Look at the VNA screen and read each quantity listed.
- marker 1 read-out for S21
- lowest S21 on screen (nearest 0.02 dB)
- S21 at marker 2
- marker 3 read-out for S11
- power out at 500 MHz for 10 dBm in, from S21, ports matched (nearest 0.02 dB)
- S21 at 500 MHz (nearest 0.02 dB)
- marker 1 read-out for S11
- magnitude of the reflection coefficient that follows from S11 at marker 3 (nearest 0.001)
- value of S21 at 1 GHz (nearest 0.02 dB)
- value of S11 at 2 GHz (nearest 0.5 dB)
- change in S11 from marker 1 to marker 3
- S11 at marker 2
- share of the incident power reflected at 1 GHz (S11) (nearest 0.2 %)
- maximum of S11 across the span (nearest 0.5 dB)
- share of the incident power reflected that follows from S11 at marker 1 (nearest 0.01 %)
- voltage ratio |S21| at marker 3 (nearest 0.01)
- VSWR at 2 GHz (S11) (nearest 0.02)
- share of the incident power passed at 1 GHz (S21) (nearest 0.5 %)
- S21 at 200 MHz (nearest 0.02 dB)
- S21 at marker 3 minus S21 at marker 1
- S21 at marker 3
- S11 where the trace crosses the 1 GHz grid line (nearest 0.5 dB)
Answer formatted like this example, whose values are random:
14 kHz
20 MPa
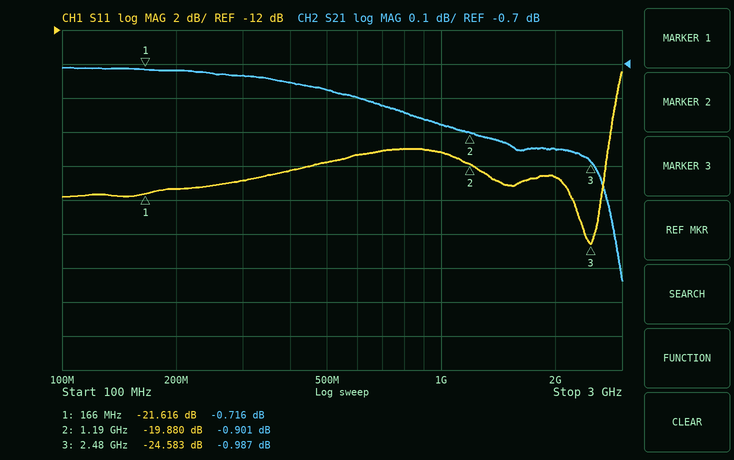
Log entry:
-0.716 dB
-1.34 dB
-0.901 dB
-24.583 dB
9.22 dBm
-0.78 dB
-21.616 dB
0.059
-0.88 dB
-20.5 dB
-2.967 dB
-19.880 dB
1.2 %
-14.5 dB
0.69 %
0.89
1.20
81.5 %
-0.72 dB
-0.271 dB
-0.987 dB
-19.0 dB
